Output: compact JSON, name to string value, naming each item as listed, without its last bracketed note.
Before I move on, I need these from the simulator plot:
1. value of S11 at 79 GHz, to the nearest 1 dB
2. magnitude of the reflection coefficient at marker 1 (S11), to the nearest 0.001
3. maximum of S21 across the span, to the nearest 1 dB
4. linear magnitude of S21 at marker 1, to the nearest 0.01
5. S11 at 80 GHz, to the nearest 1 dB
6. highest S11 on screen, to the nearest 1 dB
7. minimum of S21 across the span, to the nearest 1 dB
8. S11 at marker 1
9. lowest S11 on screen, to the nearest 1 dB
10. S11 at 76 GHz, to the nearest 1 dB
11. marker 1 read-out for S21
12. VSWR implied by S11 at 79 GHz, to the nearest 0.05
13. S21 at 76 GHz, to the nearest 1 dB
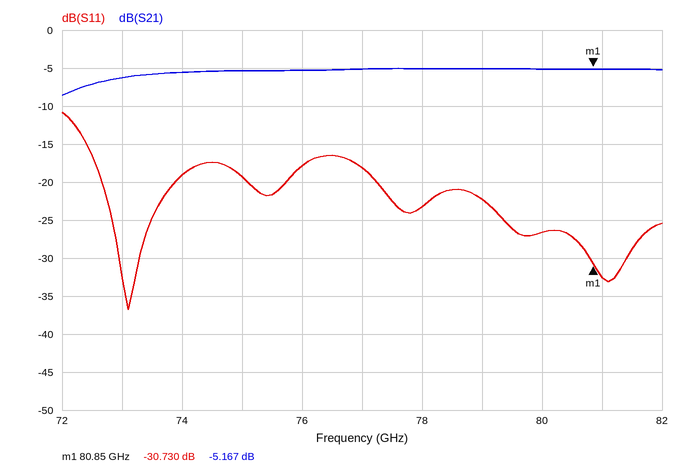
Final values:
{"value of S11 at 79 GHz, to the nearest 1 dB": "-22 dB", "magnitude of the reflection coefficient at marker 1 (S11), to the nearest 0.001": "0.029", "maximum of S21 across the span, to the nearest 1 dB": "-5 dB", "linear magnitude of S21 at marker 1, to the nearest 0.01": "0.55", "S11 at 80 GHz, to the nearest 1 dB": "-27 dB", "highest S11 on screen, to the nearest 1 dB": "-11 dB", "minimum of S21 across the span, to the nearest 1 dB": "-9 dB", "S11 at marker 1": "-30.730 dB", "lowest S11 on screen, to the nearest 1 dB": "-37 dB", "S11 at 76 GHz, to the nearest 1 dB": "-18 dB", "marker 1 read-out for S21": "-5.167 dB", "VSWR implied by S11 at 79 GHz, to the nearest 0.05": "1.15", "S21 at 76 GHz, to the nearest 1 dB": "-5 dB"}
